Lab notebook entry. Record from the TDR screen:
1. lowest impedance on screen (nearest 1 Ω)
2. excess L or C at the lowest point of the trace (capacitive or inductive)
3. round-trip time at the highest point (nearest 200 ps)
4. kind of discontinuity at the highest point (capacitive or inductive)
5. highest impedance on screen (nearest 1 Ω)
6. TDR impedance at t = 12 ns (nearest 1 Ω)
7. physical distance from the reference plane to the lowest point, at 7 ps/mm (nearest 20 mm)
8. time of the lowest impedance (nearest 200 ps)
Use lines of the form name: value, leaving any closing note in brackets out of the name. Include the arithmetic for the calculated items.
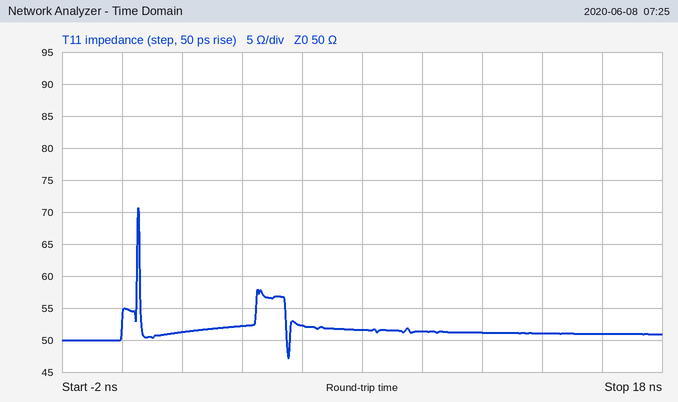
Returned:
lowest impedance on screen: 47 Ω
excess L or C at the lowest point of the trace: capacitive
round-trip time at the highest point: 600 ps
kind of discontinuity at the highest point: inductive
highest impedance on screen: 71 Ω
TDR impedance at t = 12 ns: 51 Ω
physical distance from the reference plane to the lowest point, at 7 ps/mm: 5.6 ns / 2 / 7 ps/mm ≈ 400 mm
time of the lowest impedance: 5.6 ns
